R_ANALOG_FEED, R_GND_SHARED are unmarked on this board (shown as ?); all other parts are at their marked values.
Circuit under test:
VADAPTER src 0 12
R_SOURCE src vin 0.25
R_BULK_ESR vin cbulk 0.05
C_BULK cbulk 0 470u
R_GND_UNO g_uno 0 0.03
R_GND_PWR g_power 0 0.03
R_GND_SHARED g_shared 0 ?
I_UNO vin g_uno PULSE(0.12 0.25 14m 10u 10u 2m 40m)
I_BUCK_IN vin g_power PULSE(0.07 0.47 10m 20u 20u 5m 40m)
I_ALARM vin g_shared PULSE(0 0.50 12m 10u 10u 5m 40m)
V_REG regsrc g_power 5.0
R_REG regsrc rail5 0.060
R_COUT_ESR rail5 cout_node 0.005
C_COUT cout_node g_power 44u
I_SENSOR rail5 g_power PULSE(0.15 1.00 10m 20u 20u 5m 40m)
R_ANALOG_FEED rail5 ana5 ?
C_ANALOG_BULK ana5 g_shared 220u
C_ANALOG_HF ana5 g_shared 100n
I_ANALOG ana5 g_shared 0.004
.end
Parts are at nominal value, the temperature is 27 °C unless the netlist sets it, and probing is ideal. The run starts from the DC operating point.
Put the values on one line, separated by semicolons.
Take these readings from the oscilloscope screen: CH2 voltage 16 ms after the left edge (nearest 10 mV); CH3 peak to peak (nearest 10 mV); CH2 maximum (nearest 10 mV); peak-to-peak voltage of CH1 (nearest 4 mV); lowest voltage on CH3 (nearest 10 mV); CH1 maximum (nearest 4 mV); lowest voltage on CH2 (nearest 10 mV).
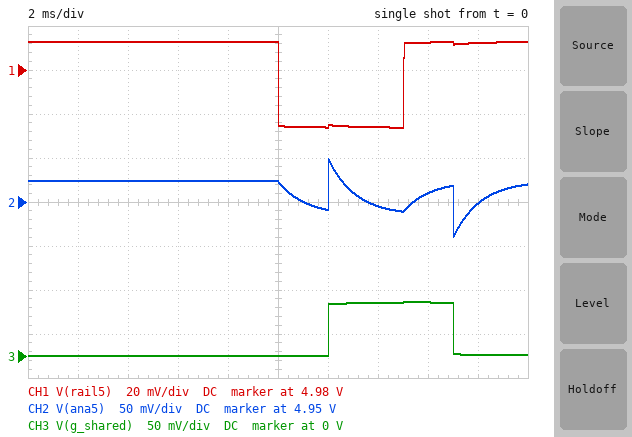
4.96 V; 60 mV; 5.00 V; 40 mV; 0 V; 4.992 V; 4.91 V
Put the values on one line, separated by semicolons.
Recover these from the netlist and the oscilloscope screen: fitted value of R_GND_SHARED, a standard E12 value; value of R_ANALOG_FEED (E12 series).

0.12 Ω; 4.7 Ω
